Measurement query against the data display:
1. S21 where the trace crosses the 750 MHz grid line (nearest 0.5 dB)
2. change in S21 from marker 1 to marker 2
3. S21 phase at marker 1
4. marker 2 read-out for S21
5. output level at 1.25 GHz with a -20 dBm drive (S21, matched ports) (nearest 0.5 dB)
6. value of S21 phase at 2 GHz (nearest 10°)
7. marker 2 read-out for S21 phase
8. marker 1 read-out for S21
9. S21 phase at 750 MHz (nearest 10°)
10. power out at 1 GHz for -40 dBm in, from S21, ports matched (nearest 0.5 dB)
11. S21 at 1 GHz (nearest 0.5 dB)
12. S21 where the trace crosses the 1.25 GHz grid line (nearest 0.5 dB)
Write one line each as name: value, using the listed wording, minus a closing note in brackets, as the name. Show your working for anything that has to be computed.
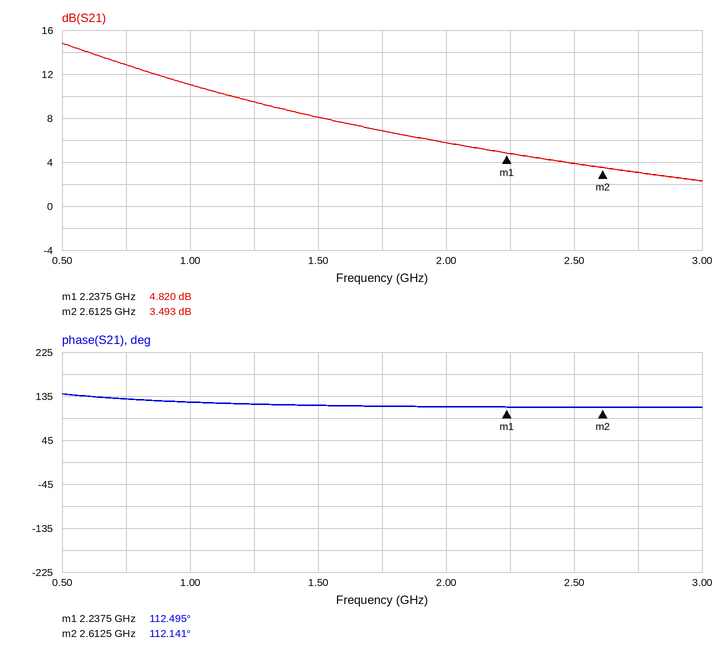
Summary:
S21 where the trace crosses the 750 MHz grid line: 13.0 dB
change in S21 from marker 1 to marker 2: 3.493 − (4.82) = -1.327 dB
S21 phase at marker 1: 112.495°
marker 2 read-out for S21: 3.493 dB
output level at 1.25 GHz with a -20 dBm drive (S21, matched ports): -20 dBm + (9.5 dB) = -10.5 dBm
value of S21 phase at 2 GHz: 110°
marker 2 read-out for S21 phase: 112.141°
marker 1 read-out for S21: 4.820 dB
S21 phase at 750 MHz: 130°
power out at 1 GHz for -40 dBm in, from S21, ports matched: -40 dBm + (11.0 dB) = -29.0 dBm
S21 at 1 GHz: 11.0 dB
S21 where the trace crosses the 1.25 GHz grid line: 9.5 dB
